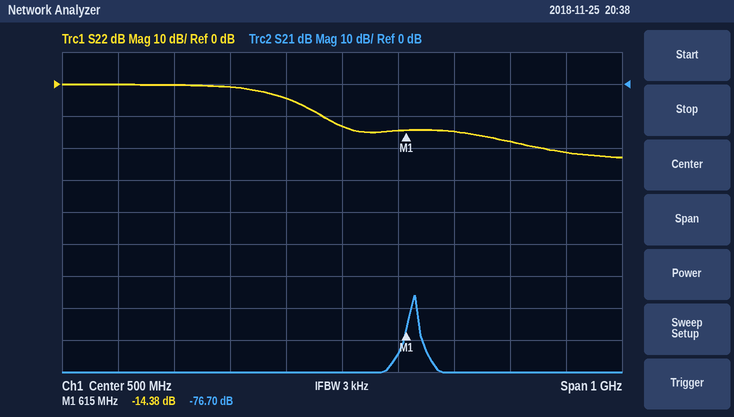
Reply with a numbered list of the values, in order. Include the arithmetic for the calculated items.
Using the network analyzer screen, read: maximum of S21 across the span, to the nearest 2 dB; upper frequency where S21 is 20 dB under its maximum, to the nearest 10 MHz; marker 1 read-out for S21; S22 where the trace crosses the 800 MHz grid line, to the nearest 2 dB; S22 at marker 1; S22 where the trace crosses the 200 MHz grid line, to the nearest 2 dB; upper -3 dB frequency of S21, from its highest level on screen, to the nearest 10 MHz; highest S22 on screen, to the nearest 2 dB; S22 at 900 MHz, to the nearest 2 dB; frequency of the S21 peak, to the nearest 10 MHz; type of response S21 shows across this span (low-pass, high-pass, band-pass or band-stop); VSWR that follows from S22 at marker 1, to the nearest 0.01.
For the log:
1. -66 dB
2. 660 MHz
3. -76.70 dB
4. -18 dB
5. -14.38 dB
6. 0 dB
7. 630 MHz
8. 0 dB
9. -22 dB
10. 630 MHz
11. band-pass
12. (1 + 0.1910)/(1 − 0.1910) ≈ 1.47
